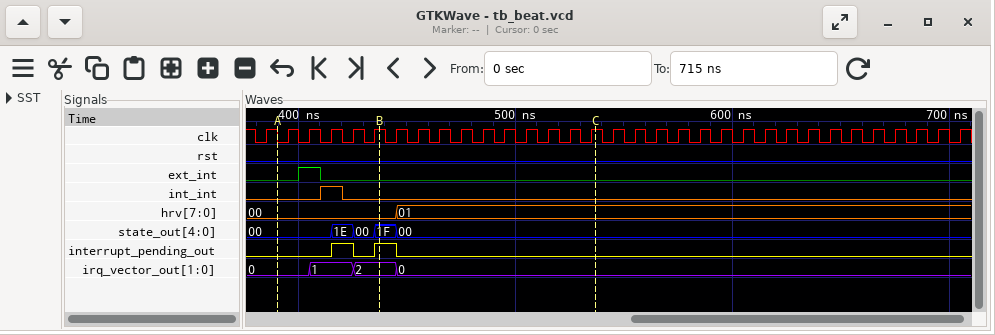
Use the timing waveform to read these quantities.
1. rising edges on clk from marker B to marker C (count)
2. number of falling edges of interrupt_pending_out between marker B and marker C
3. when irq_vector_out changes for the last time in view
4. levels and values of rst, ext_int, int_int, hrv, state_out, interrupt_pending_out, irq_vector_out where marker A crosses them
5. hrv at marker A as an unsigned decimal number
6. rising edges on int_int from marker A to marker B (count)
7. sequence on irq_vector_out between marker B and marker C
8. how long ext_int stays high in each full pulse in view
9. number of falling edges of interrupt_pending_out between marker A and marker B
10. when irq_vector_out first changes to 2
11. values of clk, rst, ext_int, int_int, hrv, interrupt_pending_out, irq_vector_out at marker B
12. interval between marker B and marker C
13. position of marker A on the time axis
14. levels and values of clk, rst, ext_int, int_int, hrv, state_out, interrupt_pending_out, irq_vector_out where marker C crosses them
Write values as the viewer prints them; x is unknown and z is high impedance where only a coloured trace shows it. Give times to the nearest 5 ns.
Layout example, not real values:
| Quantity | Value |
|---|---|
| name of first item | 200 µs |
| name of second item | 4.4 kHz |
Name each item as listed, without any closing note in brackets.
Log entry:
| Quantity | Value |
|---|---|
| rising edges on clk from marker B to marker C | 10 |
| number of falling edges of interrupt_pending_out between marker B and marker C | 1 |
| when irq_vector_out changes for the last time in view | 445 ns |
| levels and values of rst, ext_int, int_int, hrv, state_out, interrupt_pending_out, irq_vector_out where marker A crosses them | rst=0, ext_int=0, int_int=0, hrv=00, state_out=00, interrupt_pending_out=0, irq_vector_out=0 |
| hrv at marker A as an unsigned decimal number | 0 |
| rising edges on int_int from marker A to marker B | 1 |
| sequence on irq_vector_out between marker B and marker C | 2, 0 |
| how long ext_int stays high in each full pulse in view | 10 ns |
| number of falling edges of interrupt_pending_out between marker A and marker B | 1 |
| when irq_vector_out first changes to 2 | 425 ns |
| values of clk, rst, ext_int, int_int, hrv, interrupt_pending_out, irq_vector_out at marker B | clk=1, rst=0, ext_int=0, int_int=0, hrv=00, interrupt_pending_out=1, irq_vector_out=2 |
| interval between marker B and marker C | 100 ns |
| position of marker A on the time axis | 390 ns |
| levels and values of clk, rst, ext_int, int_int, hrv, state_out, interrupt_pending_out, irq_vector_out where marker C crosses them | clk=1, rst=0, ext_int=0, int_int=0, hrv=01, state_out=00, interrupt_pending_out=0, irq_vector_out=0 |
